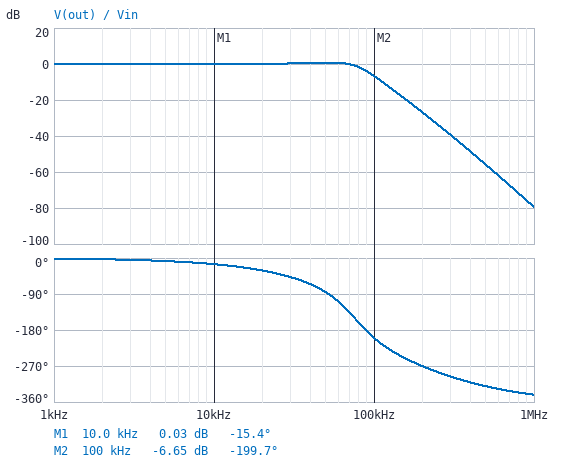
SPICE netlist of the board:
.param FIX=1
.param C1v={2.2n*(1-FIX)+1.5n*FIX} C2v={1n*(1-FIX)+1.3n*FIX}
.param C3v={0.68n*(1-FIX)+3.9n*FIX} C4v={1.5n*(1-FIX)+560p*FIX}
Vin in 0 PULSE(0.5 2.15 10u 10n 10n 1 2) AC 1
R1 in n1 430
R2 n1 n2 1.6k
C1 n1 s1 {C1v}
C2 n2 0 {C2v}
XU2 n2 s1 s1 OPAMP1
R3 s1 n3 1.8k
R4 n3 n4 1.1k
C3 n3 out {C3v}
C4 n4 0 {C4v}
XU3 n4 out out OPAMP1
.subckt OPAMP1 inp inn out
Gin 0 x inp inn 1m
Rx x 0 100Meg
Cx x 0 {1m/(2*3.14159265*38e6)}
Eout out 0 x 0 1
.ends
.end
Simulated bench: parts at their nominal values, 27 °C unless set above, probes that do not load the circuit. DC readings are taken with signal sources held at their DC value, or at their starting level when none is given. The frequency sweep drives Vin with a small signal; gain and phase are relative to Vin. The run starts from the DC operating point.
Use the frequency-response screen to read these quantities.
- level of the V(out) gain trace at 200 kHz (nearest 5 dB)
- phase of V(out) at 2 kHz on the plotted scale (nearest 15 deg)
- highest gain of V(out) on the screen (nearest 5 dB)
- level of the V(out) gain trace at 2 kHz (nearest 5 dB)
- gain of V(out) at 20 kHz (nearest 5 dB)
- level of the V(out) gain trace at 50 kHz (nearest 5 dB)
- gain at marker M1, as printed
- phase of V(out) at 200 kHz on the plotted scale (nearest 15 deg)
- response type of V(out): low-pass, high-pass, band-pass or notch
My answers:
-25 dB
0 deg
0 dB
0 dB
0 dB
0 dB
0.03 dB
-270 deg
low-pass
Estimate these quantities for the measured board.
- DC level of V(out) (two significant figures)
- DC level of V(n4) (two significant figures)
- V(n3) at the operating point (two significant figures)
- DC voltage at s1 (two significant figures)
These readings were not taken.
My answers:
500 mV
500 mV
500 mV
500 mV
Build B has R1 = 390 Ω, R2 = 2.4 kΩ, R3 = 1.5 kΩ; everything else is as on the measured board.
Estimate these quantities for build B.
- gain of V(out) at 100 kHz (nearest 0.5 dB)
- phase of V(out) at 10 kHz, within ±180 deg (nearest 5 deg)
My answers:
-7.5 dB
-20 deg
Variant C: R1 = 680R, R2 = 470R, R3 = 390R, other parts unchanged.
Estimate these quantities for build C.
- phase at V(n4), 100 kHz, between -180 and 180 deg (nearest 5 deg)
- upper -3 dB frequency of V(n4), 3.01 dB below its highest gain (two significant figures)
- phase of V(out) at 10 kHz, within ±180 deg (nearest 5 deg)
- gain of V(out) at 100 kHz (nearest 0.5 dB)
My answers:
-90 deg
170 kHz
-10 deg
0 dB
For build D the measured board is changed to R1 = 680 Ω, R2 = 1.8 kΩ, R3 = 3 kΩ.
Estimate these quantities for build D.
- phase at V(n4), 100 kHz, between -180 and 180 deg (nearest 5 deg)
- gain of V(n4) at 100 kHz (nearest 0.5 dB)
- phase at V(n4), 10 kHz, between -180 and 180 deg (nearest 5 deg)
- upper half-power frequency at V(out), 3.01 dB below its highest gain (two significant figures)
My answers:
130 deg
-13.5 dB
-20 deg
63 kHz
